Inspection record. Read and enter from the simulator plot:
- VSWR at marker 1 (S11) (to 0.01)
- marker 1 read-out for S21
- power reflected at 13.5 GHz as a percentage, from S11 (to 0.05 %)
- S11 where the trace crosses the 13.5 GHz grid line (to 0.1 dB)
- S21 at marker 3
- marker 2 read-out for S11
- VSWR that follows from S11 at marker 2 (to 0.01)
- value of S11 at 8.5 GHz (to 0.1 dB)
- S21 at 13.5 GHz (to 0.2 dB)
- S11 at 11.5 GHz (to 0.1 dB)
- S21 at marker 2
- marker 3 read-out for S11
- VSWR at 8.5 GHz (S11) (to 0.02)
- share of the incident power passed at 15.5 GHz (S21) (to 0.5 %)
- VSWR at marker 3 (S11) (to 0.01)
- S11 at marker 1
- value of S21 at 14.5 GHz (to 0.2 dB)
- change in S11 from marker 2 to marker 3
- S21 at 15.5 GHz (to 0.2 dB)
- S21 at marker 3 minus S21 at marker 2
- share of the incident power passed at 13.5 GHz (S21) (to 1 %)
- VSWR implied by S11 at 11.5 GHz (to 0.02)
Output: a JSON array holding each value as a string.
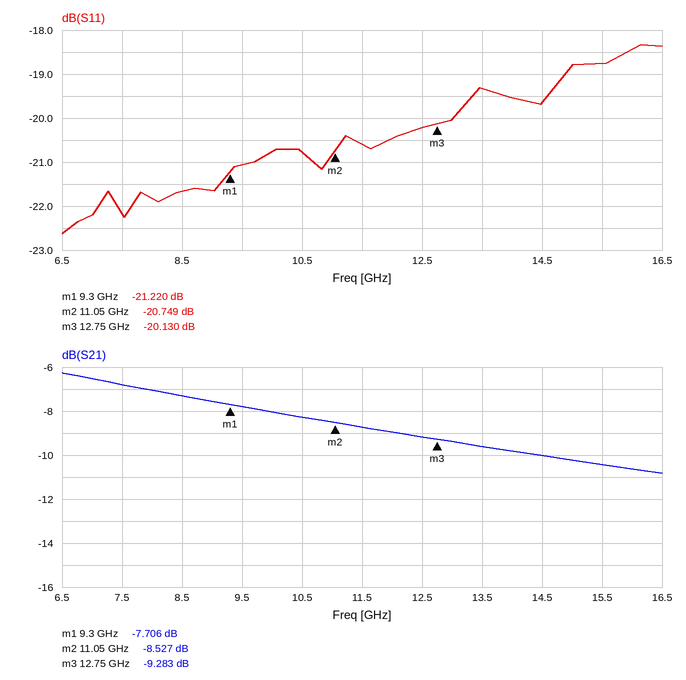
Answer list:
["1.19", "-7.706 dB", "1.15 %", "-19.3 dB", "-9.283 dB", "-20.749 dB", "1.20", "-21.7 dB", "-9.6 dB", "-20.6 dB", "-8.527 dB", "-20.130 dB", "1.18", "9.0 %", "1.22", "-21.220 dB", "-10.0 dB", "0.619 dB", "-10.4 dB", "-0.756 dB", "11 %", "1.20"]
